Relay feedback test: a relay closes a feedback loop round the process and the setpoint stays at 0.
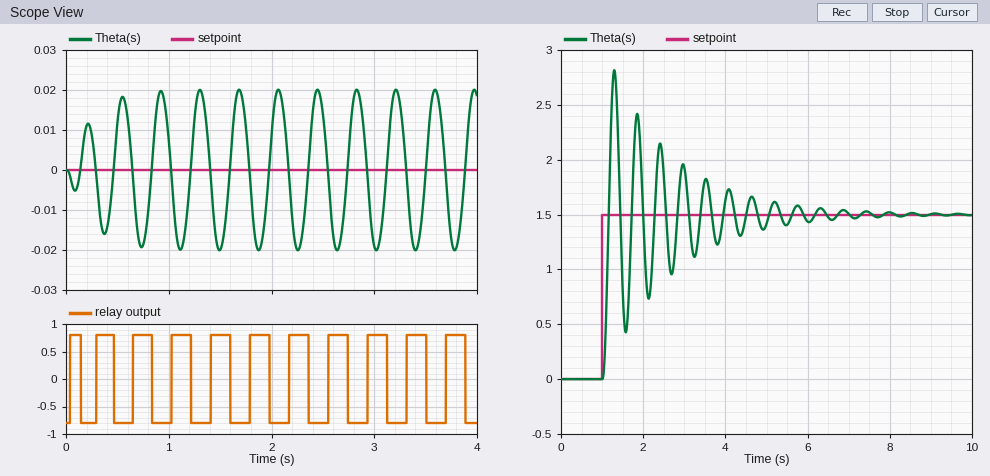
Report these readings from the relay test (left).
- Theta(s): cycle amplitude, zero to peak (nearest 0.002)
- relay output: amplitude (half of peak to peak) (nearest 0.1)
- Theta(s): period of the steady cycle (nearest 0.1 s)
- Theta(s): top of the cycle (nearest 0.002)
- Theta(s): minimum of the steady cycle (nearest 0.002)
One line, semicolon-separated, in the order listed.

0.020; 0.8; 0.4 s; 0.020; -0.020
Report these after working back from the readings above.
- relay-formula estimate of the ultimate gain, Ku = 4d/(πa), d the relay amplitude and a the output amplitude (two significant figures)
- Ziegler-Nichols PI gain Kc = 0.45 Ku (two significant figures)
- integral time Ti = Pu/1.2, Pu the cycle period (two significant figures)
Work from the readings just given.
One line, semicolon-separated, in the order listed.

51; 23; 0.33 s
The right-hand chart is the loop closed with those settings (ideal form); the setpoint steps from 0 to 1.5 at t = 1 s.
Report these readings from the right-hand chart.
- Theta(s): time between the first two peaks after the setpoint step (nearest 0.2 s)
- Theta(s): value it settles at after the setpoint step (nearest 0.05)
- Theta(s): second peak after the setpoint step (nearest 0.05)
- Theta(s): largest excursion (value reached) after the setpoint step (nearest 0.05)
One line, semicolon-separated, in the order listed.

0.6 s; 1.50; 2.40; 2.80
